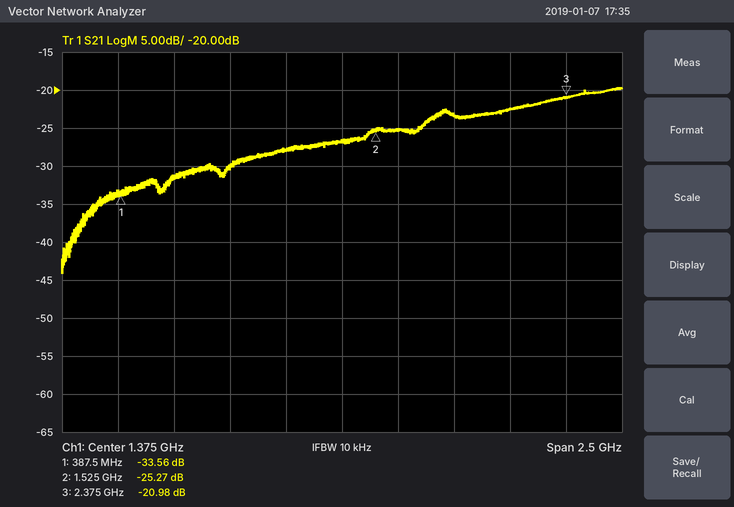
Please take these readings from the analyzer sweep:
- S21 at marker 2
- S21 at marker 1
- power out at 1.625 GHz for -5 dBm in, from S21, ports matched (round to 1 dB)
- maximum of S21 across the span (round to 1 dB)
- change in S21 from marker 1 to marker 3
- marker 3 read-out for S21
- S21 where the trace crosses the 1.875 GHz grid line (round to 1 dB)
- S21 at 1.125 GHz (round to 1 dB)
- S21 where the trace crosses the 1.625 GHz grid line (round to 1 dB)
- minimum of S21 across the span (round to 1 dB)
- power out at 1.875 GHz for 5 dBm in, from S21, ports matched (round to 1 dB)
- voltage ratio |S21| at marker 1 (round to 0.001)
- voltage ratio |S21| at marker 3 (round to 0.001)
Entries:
-25.27 dB
-33.56 dB
-30 dBm
-20 dB
12.58 dB
-20.98 dB
-23 dB
-28 dB
-25 dB
-44 dB
-18 dBm
0.021
0.089
